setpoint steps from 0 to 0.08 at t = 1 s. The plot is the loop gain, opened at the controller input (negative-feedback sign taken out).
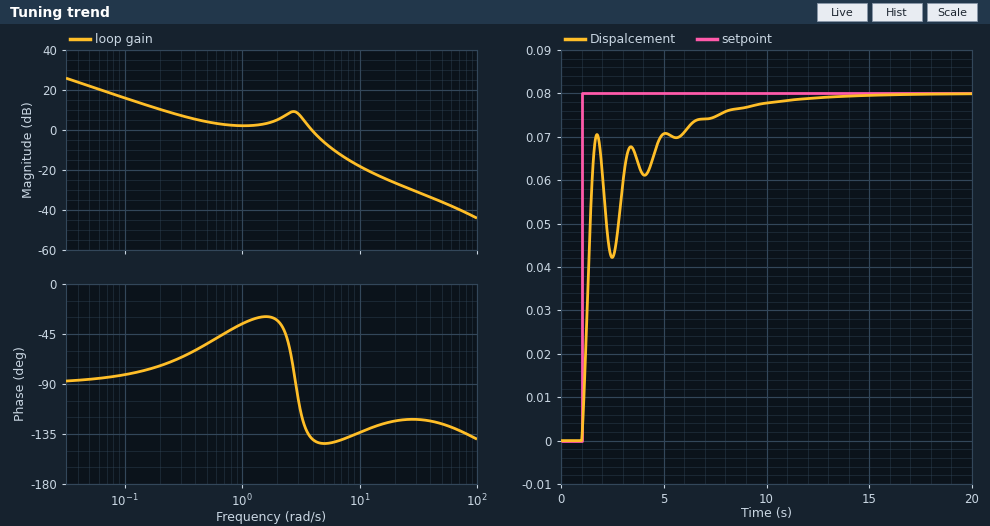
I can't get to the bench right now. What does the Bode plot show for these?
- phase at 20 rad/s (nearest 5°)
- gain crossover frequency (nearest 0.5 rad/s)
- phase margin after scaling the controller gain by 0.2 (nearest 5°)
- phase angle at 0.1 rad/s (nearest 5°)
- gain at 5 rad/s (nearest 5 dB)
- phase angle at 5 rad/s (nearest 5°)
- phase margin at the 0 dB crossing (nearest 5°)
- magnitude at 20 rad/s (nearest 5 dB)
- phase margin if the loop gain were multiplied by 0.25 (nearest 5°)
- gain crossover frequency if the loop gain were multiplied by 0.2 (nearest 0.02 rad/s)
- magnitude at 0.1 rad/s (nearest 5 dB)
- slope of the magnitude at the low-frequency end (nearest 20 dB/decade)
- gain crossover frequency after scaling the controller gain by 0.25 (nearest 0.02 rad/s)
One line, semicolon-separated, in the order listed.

-125°; 4.0 rad/s; 100°; -80°; -5 dB; -145°; 40°; -25 dB; 105°; 0.12 rad/s; 15 dB; -20 dB/decade; 0.16 rad/s
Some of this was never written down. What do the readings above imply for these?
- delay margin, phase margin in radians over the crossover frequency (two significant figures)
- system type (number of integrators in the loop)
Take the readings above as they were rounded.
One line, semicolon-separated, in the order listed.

0.17 s; 1
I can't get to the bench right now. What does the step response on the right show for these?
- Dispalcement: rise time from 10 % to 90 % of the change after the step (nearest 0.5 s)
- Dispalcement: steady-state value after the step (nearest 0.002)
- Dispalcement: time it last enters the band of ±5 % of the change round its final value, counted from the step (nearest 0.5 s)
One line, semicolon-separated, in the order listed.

5.0 s; 0.080; 7.0 s
